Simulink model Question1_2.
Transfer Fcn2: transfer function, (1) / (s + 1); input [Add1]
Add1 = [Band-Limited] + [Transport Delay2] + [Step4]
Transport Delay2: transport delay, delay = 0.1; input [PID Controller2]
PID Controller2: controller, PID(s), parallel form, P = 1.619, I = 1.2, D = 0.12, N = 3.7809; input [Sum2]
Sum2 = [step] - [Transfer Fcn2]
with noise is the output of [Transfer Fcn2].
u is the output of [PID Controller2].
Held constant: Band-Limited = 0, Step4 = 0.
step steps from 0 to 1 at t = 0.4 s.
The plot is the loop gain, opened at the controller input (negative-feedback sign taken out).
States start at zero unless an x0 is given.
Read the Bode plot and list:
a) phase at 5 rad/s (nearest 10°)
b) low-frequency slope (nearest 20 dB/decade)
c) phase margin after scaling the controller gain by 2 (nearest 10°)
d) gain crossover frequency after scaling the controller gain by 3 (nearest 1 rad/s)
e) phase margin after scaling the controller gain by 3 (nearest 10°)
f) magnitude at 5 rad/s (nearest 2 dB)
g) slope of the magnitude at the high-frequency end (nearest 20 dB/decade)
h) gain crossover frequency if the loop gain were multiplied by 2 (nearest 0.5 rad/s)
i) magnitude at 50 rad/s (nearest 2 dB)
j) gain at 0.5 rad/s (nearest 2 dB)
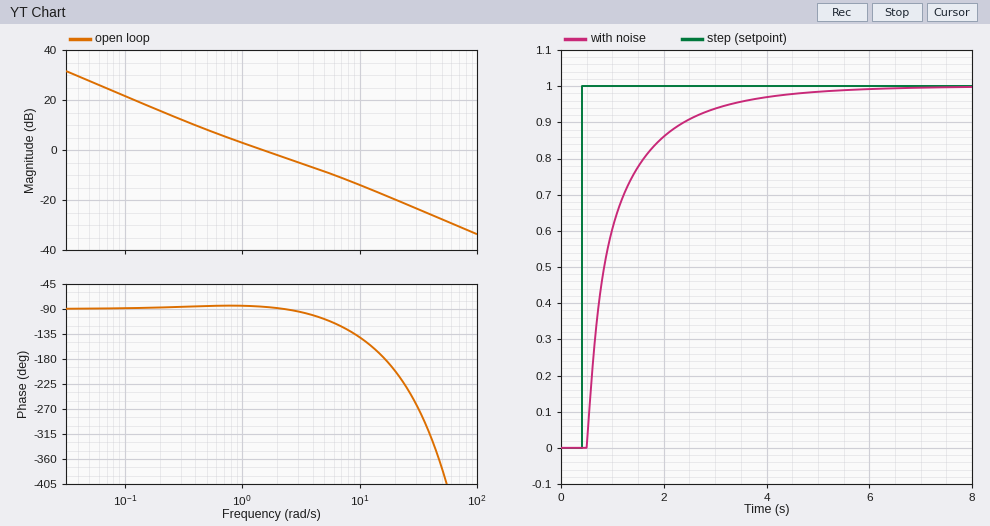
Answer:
-110°
-20 dB/decade
80°
6 rad/s
70°
-8 dB
-20 dB/decade
3.5 rad/s
-28 dB
8 dB
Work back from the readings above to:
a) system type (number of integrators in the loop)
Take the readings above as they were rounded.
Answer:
1
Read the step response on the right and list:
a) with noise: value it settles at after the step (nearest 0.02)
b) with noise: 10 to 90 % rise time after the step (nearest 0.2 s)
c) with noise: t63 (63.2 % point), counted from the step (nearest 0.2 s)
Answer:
1.00
1.8 s
0.6 s
